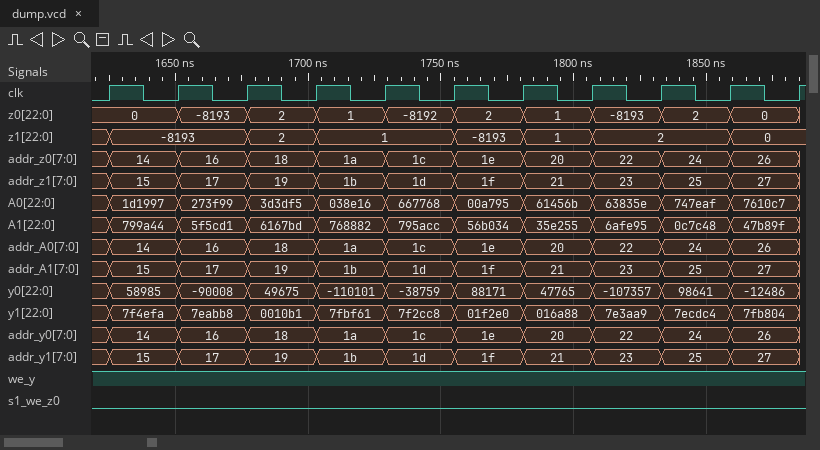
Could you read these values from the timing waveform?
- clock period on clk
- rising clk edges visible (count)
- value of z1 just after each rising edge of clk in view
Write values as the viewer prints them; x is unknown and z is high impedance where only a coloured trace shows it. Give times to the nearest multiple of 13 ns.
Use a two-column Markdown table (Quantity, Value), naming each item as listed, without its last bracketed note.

| Quantity | Value |
|---|---|
| clock period on clk | 26 ns |
| rising clk edges visible | 11 |
| value of z1 just after each rising edge of clk in view | -8193, -8193, 2, 1, 1, -8193, 1, 2, 2, 0, 0 |
